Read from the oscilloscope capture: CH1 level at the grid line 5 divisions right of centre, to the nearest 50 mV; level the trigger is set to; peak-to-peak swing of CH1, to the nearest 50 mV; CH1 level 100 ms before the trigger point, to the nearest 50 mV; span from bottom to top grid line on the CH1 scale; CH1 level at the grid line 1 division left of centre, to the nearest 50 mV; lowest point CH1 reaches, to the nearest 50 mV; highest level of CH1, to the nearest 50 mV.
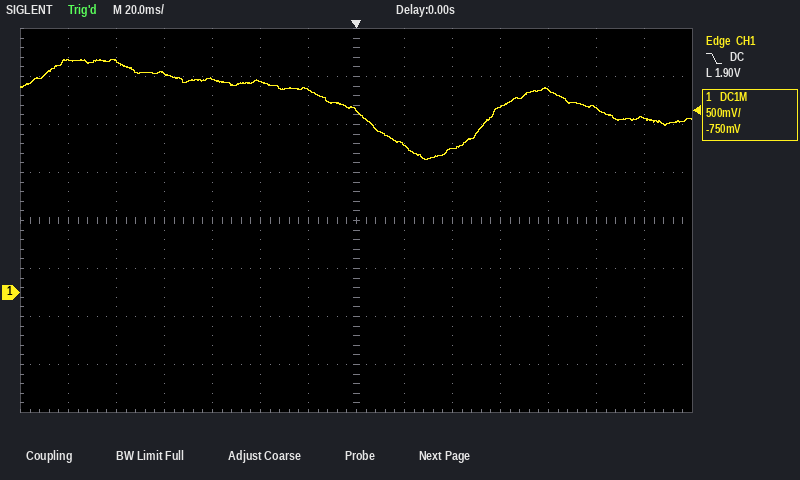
1.90 V
1.90 V
1.05 V
2.40 V
4 V
2.10 V
1.40 V
2.45 V
